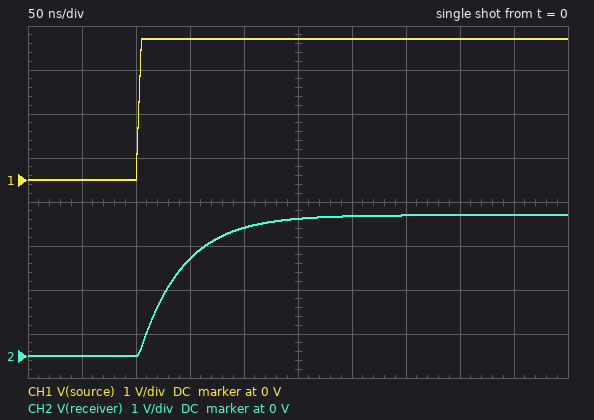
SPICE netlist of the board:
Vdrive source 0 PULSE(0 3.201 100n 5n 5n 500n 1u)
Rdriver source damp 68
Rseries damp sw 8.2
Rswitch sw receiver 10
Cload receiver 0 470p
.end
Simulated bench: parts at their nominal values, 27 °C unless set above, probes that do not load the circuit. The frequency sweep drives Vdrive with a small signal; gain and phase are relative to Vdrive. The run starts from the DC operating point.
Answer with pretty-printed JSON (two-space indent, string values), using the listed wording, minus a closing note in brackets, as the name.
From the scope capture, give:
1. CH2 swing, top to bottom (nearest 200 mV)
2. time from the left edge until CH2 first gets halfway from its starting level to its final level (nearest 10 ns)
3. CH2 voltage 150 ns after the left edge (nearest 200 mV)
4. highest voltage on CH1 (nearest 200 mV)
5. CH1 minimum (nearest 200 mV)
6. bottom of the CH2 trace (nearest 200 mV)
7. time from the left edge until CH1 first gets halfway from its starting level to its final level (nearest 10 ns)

{
  "CH2 swing, top to bottom": "3.2 V",
  "time from the left edge until CH2 first gets halfway from its starting level to its final level": "130 ns",
  "CH2 voltage 150 ns after the left edge": "2.2 V",
  "highest voltage on CH1": "3.2 V",
  "CH1 minimum": "0 V",
  "bottom of the CH2 trace": "0 V",
  "time from the left edge until CH1 first gets halfway from its starting level to its final level": "100 ns"
}
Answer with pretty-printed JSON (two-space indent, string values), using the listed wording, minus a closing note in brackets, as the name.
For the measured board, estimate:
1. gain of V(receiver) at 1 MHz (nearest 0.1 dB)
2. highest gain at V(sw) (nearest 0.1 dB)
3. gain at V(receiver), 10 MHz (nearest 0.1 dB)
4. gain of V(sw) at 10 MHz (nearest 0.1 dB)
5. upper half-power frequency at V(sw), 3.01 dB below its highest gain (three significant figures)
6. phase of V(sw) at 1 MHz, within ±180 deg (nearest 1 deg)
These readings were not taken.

{
  "gain of V(receiver) at 1 MHz": "-0.3 dB",
  "highest gain at V(sw)": "0 dB",
  "gain at V(receiver), 10 MHz": "-8.7 dB",
  "gain of V(sw) at 10 MHz": "-8.4 dB",
  "upper half-power frequency at V(sw), 3.01 dB below its highest gain": "3.98 MHz",
  "phase of V(sw) at 1 MHz, within ±180 deg": "-13 deg"
}
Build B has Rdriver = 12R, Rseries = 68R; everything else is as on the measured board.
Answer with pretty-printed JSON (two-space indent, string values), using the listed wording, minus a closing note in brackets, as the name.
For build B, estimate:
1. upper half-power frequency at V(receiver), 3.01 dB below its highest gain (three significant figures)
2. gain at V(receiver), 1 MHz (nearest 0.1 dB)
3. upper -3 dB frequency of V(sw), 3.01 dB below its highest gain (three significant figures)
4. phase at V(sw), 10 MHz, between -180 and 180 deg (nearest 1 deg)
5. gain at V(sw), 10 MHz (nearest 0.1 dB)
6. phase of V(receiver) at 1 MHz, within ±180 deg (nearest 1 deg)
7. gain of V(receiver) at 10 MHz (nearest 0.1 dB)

{
  "upper half-power frequency at V(receiver), 3.01 dB below its highest gain": "3.76 MHz",
  "gain at V(receiver), 1 MHz": "-0.3 dB",
  "upper -3 dB frequency of V(sw), 3.01 dB below its highest gain": "3.81 MHz",
  "phase at V(sw), 10 MHz, between -180 and 180 deg": "-53 deg",
  "gain at V(sw), 10 MHz": "-8.7 dB",
  "phase of V(receiver) at 1 MHz, within ±180 deg": "-15 deg",
  "gain of V(receiver) at 10 MHz": "-9.1 dB"
}
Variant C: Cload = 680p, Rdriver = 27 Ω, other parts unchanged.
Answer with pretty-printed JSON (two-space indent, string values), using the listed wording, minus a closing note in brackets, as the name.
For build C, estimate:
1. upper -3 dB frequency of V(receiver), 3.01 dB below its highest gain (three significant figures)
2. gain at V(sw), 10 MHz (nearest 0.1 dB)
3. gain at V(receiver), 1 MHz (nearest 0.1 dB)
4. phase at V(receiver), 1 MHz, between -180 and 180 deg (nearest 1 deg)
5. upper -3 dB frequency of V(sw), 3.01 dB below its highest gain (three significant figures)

{
  "upper -3 dB frequency of V(receiver), 3.01 dB below its highest gain": "5.18 MHz",
  "gain at V(sw), 10 MHz": "-6.0 dB",
  "gain at V(receiver), 1 MHz": "-0.2 dB",
  "phase at V(receiver), 1 MHz, between -180 and 180 deg": "-11 deg",
  "upper -3 dB frequency of V(sw), 3.01 dB below its highest gain": "5.45 MHz"
}
